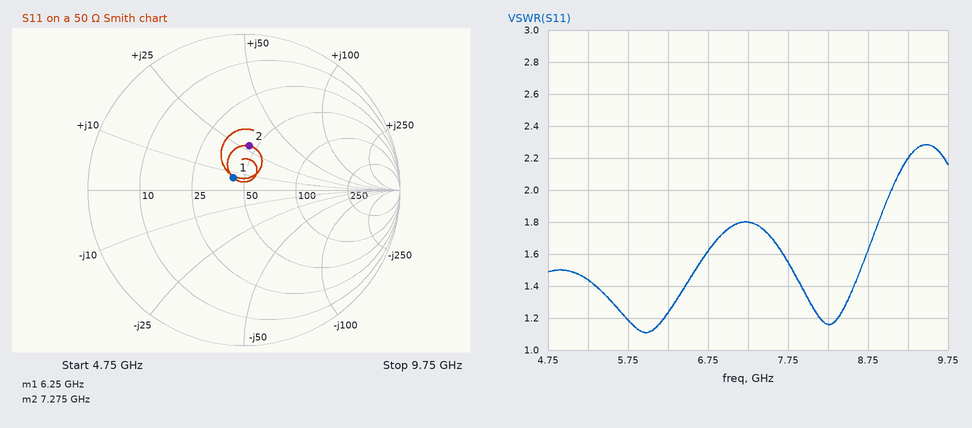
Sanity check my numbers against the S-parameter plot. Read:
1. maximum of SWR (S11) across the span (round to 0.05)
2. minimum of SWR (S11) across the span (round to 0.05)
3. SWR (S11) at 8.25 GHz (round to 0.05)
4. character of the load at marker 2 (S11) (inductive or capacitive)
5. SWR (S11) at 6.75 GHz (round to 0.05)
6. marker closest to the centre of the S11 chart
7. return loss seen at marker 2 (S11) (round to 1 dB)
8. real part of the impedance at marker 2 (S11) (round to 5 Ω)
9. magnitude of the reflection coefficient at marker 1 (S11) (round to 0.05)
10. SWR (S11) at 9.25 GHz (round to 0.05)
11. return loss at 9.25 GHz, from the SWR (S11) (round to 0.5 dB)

2.30
1.10
1.15
inductive
1.60
marker 1
11 dB
45 Ω
0.10
2.20
8.5 dB
